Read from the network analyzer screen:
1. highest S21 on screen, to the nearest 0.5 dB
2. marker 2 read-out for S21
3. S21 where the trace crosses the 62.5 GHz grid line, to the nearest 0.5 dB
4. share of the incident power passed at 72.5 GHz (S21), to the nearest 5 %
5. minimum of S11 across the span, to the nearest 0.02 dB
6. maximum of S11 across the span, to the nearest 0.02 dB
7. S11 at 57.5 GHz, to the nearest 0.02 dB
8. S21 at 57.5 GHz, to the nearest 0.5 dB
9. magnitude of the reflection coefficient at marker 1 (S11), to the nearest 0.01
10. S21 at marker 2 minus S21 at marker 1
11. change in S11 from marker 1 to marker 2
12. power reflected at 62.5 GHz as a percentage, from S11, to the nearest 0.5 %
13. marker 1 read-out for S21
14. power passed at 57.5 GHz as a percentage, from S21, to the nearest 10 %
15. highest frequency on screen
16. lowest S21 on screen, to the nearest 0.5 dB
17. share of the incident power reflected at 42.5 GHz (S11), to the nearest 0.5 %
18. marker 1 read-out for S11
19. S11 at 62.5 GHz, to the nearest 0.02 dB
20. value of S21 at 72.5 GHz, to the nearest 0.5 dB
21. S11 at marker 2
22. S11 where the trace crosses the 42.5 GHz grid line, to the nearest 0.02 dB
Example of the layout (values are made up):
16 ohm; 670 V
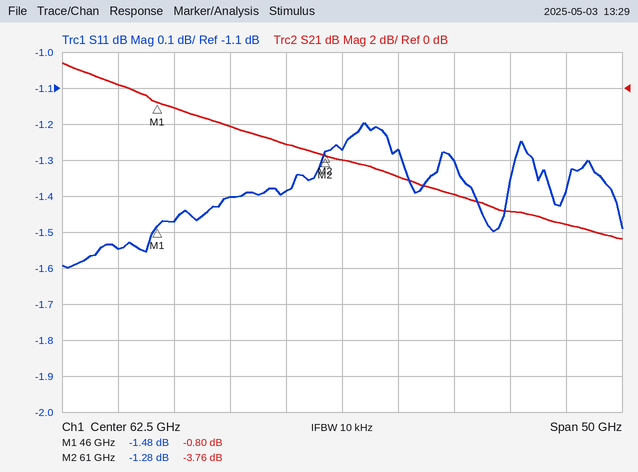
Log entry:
1.5 dB; -3.76 dB; -4.0 dB; 25 %; -1.60 dB; -1.20 dB; -1.38 dB; -3.0 dB; 0.84; -2.96 dB; 0.20 dB; 74.5 %; -0.80 dB; 50 %; 87.5 GHz; -8.5 dB; 70.0 %; -1.48 dB; -1.28 dB; -6.0 dB; -1.28 dB; -1.54 dB
